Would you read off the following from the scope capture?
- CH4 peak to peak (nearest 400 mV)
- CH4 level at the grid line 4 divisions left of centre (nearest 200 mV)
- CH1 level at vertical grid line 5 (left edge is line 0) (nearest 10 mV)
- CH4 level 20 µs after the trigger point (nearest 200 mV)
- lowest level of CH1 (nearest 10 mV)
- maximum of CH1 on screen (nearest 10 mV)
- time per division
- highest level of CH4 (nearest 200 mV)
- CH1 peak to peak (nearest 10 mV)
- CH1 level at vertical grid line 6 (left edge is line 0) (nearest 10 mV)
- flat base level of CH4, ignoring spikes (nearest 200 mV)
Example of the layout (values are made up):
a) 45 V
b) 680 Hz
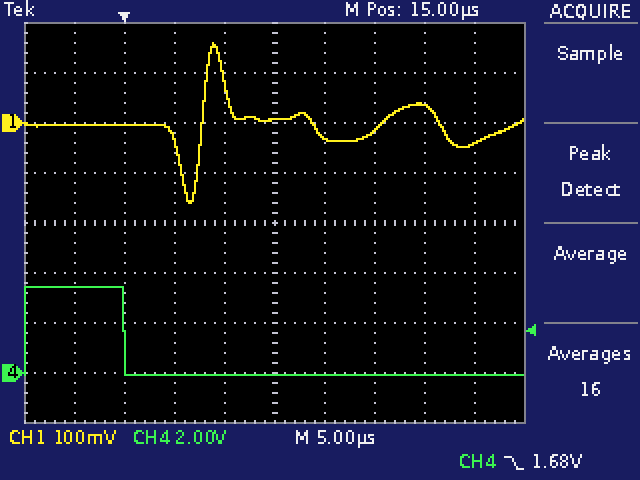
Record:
a) 3.6 V
b) 3.4 V
c) 10 mV
d) 0.0 V
e) -160 mV
f) 160 mV
g) 5 µs
h) 3.4 V
i) 320 mV
j) -30 mV
k) 0.0 V
